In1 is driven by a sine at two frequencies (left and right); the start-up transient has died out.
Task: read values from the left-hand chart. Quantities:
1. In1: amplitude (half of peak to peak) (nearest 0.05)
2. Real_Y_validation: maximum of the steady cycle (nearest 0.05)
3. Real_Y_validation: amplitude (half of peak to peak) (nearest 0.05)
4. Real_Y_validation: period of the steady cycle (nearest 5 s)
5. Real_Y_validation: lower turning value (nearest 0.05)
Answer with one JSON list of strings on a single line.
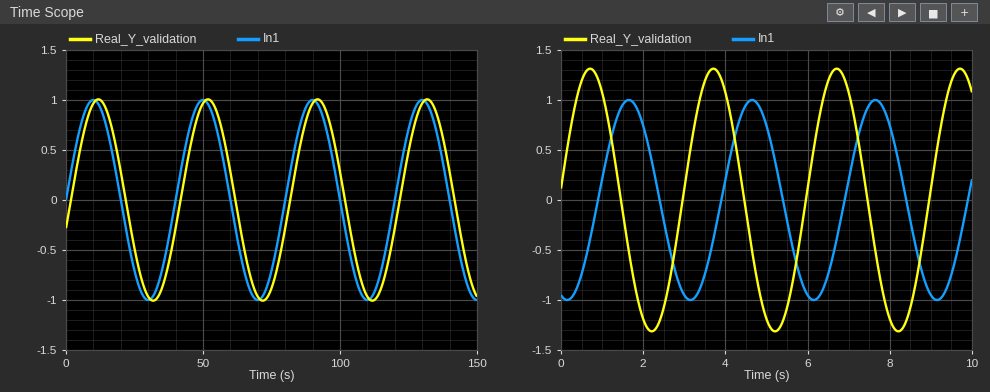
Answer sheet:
["1.00", "1.00", "1.00", "40 s", "-1.00"]
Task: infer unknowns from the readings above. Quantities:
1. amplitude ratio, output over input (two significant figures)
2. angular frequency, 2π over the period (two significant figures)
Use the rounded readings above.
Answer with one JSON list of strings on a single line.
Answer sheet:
["1.0", "0.16 rad/s"]
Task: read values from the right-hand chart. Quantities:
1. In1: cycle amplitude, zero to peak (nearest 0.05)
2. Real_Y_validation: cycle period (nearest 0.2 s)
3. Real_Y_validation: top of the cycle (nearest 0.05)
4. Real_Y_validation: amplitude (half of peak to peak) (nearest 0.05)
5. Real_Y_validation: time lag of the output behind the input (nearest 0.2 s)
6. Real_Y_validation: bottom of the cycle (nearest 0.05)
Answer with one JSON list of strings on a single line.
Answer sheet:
["1.00", "3.0 s", "1.30", "1.30", "2.0 s", "-1.30"]
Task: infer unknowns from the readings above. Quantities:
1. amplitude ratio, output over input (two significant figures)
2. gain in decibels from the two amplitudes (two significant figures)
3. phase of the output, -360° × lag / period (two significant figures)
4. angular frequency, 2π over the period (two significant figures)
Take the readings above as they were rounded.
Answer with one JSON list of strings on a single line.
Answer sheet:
["1.3", "2.3 dB", "-240°", "2.1 rad/s"]
